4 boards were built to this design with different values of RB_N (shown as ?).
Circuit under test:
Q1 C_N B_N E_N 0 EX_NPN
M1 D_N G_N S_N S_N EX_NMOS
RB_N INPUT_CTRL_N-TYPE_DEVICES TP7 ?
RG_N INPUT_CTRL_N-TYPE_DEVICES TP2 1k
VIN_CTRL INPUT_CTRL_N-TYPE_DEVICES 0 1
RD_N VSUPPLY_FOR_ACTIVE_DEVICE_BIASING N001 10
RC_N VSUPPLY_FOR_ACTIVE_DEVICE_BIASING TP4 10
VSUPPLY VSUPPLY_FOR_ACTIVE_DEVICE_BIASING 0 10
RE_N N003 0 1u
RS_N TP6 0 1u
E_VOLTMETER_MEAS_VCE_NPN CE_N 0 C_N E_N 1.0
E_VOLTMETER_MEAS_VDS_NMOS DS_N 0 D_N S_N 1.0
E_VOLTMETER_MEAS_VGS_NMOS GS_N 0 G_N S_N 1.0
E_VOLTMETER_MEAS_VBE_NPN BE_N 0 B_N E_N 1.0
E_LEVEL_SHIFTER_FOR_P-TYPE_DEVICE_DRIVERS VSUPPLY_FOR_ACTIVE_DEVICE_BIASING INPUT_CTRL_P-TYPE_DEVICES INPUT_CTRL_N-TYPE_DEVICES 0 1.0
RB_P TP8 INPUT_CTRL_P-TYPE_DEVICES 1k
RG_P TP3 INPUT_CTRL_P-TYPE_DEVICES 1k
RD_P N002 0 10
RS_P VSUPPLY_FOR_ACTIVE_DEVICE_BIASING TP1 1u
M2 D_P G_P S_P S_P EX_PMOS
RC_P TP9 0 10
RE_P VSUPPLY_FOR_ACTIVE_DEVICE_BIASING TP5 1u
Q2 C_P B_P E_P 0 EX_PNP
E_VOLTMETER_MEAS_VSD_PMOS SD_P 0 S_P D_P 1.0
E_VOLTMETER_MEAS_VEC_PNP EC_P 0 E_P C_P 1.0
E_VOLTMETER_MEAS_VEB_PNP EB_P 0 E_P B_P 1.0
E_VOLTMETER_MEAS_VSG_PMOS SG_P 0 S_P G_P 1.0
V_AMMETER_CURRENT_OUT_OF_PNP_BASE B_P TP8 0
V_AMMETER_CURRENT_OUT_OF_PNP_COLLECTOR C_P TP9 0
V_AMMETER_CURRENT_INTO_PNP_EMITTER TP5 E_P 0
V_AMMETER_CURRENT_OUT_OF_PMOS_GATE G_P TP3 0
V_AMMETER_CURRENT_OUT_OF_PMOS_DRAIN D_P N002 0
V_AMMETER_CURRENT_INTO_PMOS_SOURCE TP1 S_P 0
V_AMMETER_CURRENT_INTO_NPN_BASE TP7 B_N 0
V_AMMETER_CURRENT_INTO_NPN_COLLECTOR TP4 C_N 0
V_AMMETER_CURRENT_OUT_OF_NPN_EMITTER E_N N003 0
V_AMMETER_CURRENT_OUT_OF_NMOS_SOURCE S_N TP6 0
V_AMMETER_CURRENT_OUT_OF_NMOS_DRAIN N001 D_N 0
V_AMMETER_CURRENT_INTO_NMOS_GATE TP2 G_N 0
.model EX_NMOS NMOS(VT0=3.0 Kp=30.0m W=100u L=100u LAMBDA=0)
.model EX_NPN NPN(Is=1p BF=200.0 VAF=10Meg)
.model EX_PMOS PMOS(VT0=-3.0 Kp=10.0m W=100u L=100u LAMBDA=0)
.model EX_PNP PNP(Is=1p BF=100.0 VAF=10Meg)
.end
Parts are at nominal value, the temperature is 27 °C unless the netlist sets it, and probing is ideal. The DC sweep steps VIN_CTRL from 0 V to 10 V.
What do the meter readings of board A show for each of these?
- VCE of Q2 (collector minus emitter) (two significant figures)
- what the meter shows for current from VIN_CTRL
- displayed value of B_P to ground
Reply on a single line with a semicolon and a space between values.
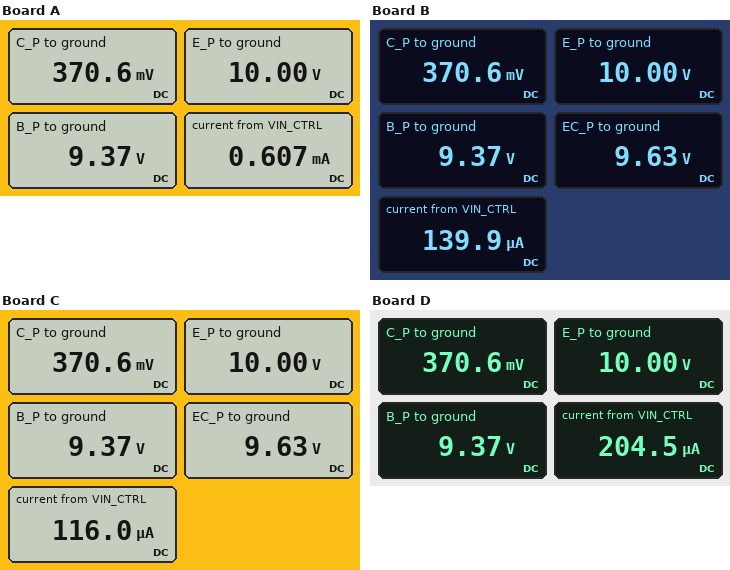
-9.6 V; 0.607 mA; 9.37 V
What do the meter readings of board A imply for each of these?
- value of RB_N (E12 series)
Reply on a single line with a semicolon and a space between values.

560 Ω
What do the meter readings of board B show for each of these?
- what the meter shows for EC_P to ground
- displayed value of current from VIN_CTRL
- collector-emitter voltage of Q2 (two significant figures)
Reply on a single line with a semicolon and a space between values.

9.63 V; 139.9 µA; -9.6 V
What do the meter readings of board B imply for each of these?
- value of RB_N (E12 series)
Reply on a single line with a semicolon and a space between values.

2.7 kΩ
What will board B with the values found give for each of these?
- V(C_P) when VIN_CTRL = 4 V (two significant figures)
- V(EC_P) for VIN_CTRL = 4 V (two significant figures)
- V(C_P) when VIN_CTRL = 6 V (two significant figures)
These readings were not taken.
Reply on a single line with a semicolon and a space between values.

3.3 V; 6.7 V; 5.3 V
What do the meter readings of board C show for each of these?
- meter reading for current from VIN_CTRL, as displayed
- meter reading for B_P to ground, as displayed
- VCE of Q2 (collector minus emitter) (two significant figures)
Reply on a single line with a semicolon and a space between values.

116.0 µA; 9.37 V; -9.6 V
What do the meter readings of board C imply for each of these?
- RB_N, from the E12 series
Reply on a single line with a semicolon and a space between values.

3.3 kΩ
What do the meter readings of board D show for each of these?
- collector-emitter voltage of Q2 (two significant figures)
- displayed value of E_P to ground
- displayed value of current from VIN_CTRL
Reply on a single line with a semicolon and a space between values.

-9.6 V; 10.00 V; 204.5 µA
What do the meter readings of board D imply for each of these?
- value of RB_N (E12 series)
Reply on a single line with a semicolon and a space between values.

1.8 kΩ
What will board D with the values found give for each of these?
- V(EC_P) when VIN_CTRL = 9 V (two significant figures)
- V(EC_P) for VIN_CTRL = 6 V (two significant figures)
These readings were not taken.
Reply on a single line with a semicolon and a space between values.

1.7 V; 4.7 V
